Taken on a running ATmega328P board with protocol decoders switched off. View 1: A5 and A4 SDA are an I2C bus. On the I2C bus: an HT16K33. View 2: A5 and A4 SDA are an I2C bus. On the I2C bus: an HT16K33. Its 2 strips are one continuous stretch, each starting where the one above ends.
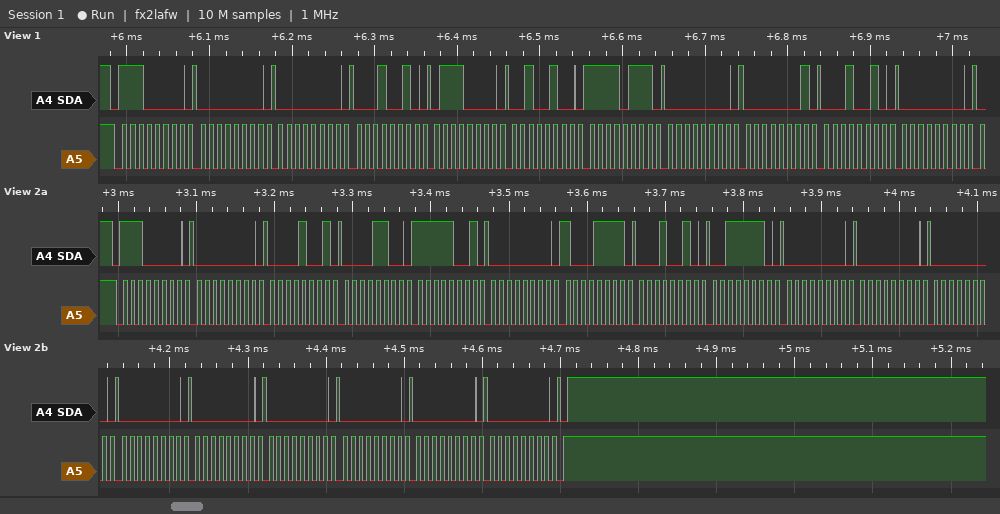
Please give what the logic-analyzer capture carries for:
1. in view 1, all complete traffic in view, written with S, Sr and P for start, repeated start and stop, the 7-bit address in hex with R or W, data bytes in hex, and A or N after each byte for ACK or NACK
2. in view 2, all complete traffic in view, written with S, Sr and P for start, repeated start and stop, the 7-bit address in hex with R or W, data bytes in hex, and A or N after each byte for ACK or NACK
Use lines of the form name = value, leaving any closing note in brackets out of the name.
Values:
in view 1, all complete traffic in view, written with S, Sr and P for start, repeated start and stop, the 7-bit address in hex with R or W, data bytes in hex, and A or N after each byte for ACK or NACK = S 70W A 00 A 00 A 12 A 70 A 24 A F7 A 00 A 01 A 12 A 00 A
in view 2, all complete traffic in view, written with S, Sr and P for start, repeated start and stop, the 7-bit address in hex with R or W, data bytes in hex, and A or N after each byte for ACK or NACK = S 70W A 00 A 09 A 0C A F9 A 00 A 8F A 12 A 3E A 00 A 00 A 00 A 00 A 00 A 00 A 00 A 00 A 00 A P
